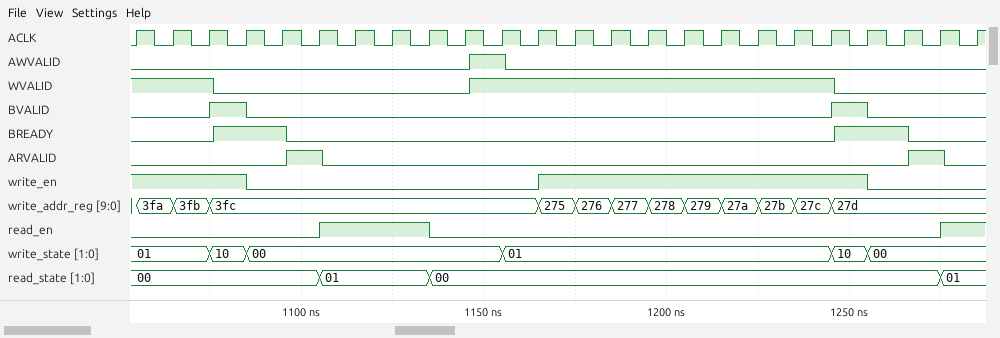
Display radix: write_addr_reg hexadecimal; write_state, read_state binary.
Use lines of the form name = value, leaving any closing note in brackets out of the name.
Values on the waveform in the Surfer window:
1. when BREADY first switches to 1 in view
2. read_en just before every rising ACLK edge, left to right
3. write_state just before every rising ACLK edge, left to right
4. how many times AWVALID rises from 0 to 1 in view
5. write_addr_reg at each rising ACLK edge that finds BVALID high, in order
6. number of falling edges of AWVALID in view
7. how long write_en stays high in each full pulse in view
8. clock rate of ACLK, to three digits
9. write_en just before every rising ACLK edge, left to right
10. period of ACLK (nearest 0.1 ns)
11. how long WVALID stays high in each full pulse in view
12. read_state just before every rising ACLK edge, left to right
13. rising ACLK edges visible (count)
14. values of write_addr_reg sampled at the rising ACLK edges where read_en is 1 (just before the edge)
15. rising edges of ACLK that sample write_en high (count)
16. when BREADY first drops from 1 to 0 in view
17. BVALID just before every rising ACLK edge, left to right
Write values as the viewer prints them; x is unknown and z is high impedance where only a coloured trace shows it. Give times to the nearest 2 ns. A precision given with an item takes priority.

when BREADY first switches to 1 in view = 1076 ns
read_en just before every rising ACLK edge, left to right = 0 0 0 0 0 0 1 1 1 0 0 0 0 0 0 0 0 0 0 0 0 0 0 1
write_state just before every rising ACLK edge, left to right = 01, 01, 01, 10, 00, 00, 00, 00, 00, 00, 00, 01, 01, 01, 01, 01, 01, 01, 01, 01, 10, 00, 00, 00
how many times AWVALID rises from 0 to 1 in view = 1
write_addr_reg at each rising ACLK edge that finds BVALID high, in order = 3fc, 27d
number of falling edges of AWVALID in view = 1
how long write_en stays high in each full pulse in view = 90 ns
clock rate of ACLK, to three digits = 100 MHz
write_en just before every rising ACLK edge, left to right = 1 1 1 1 0 0 0 0 0 0 0 0 1 1 1 1 1 1 1 1 1 0 0 0
period of ACLK = 10 ns
how long WVALID stays high in each full pulse in view = 100 ns
read_state just before every rising ACLK edge, left to right = 00, 00, 00, 00, 00, 00, 01, 01, 01, 00, 00, 00, 00, 00, 00, 00, 00, 00, 00, 00, 00, 00, 00, 01
rising ACLK edges visible = 24
values of write_addr_reg sampled at the rising ACLK edges where read_en is 1 = 3fc, 3fc, 3fc, 27d
rising edges of ACLK that sample write_en high = 13
when BREADY first drops from 1 to 0 in view = 1096 ns
BVALID just before every rising ACLK edge, left to right = 0 0 0 1 0 0 0 0 0 0 0 0 0 0 0 0 0 0 0 0 1 0 0 0
